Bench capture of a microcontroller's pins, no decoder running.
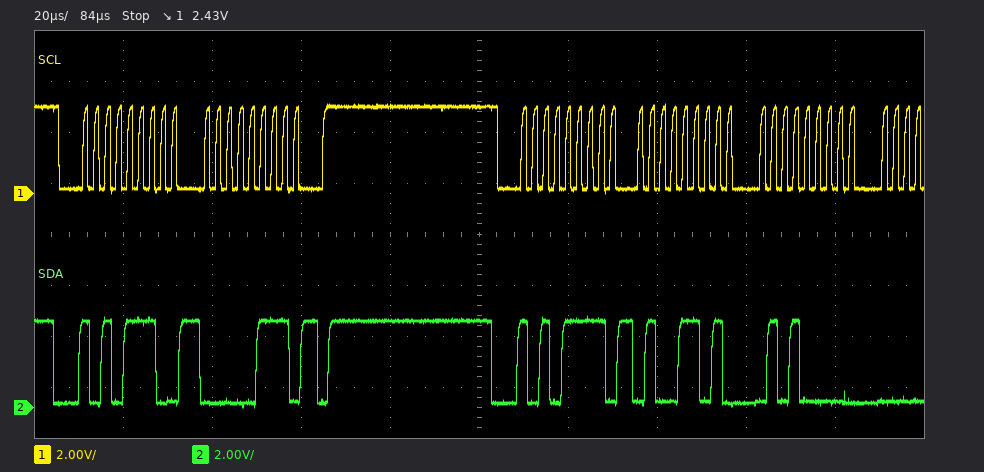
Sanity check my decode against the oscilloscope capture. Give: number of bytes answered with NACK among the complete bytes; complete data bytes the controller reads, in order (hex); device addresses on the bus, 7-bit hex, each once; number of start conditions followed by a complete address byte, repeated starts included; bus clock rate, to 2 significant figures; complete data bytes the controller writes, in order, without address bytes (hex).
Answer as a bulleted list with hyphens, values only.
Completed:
- 0
- 4D 50
- 0x57
- 2
- 400 kHz
- 07
